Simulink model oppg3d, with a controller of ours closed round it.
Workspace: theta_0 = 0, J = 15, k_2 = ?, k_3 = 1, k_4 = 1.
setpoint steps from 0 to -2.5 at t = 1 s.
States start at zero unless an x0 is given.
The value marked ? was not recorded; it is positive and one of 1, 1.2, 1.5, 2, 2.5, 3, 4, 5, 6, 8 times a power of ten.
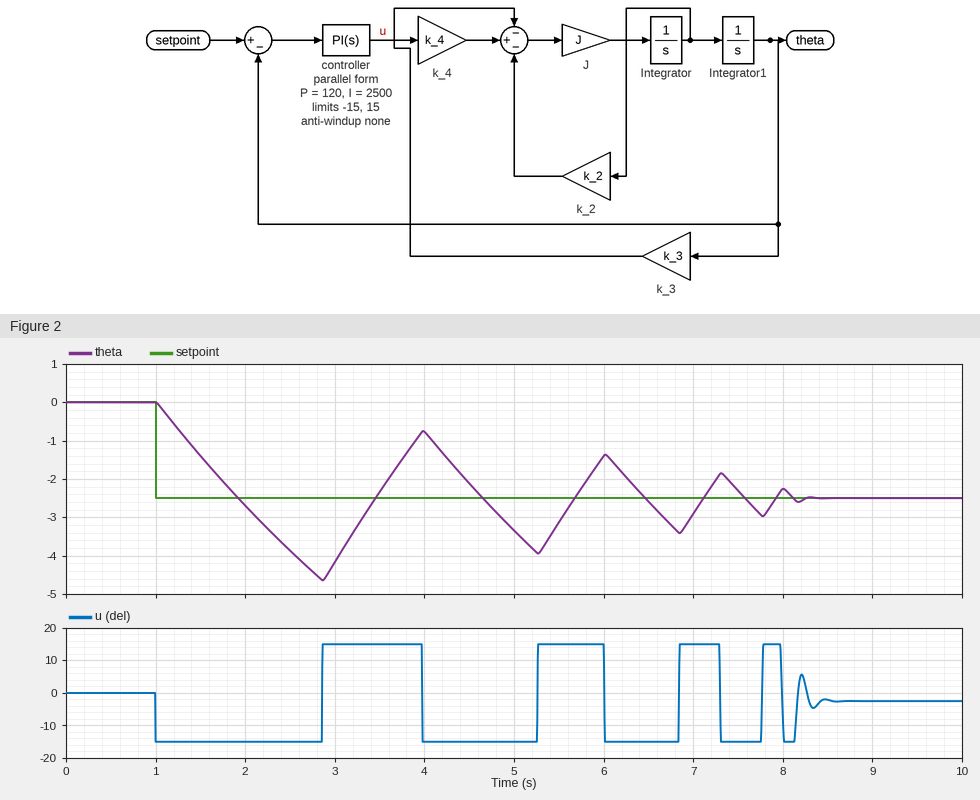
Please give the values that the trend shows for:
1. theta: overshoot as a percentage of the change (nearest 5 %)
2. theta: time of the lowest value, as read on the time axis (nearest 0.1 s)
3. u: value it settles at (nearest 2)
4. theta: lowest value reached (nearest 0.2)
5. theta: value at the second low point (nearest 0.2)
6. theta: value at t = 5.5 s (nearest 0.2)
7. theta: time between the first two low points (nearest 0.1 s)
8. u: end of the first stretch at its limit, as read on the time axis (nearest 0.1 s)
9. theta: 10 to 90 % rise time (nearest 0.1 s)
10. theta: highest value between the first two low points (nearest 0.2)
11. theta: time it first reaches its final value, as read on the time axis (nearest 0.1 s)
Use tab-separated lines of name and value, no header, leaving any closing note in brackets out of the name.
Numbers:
theta: overshoot as a percentage of the change	85 %
theta: time of the lowest value, as read on the time axis	2.9 s
u: value it settles at	-2
theta: lowest value reached	-4.6
theta: value at the second low point	-4.0
theta: value at t = 5.5 s	-3.2
theta: time between the first two low points	2.4 s
u: end of the first stretch at its limit, as read on the time axis	2.9 s
theta: 10 to 90 % rise time	0.7 s
theta: highest value between the first two low points	-0.8
theta: time it first reaches its final value, as read on the time axis	1.9 s
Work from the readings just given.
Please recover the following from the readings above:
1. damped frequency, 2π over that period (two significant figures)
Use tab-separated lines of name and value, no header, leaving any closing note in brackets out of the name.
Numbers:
damped frequency, 2π over that period	2.6 rad/s
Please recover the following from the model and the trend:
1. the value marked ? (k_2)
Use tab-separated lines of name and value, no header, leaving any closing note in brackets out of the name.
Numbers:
the value marked ?	5
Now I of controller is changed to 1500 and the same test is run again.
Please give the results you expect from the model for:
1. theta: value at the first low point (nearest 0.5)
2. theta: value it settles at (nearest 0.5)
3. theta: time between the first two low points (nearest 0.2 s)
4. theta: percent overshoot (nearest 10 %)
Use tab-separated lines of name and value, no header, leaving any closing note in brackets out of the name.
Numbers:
theta: value at the first low point	-4.5
theta: value it settles at	-2.5
theta: time between the first two low points	2.0 s
theta: percent overshoot	80 %
